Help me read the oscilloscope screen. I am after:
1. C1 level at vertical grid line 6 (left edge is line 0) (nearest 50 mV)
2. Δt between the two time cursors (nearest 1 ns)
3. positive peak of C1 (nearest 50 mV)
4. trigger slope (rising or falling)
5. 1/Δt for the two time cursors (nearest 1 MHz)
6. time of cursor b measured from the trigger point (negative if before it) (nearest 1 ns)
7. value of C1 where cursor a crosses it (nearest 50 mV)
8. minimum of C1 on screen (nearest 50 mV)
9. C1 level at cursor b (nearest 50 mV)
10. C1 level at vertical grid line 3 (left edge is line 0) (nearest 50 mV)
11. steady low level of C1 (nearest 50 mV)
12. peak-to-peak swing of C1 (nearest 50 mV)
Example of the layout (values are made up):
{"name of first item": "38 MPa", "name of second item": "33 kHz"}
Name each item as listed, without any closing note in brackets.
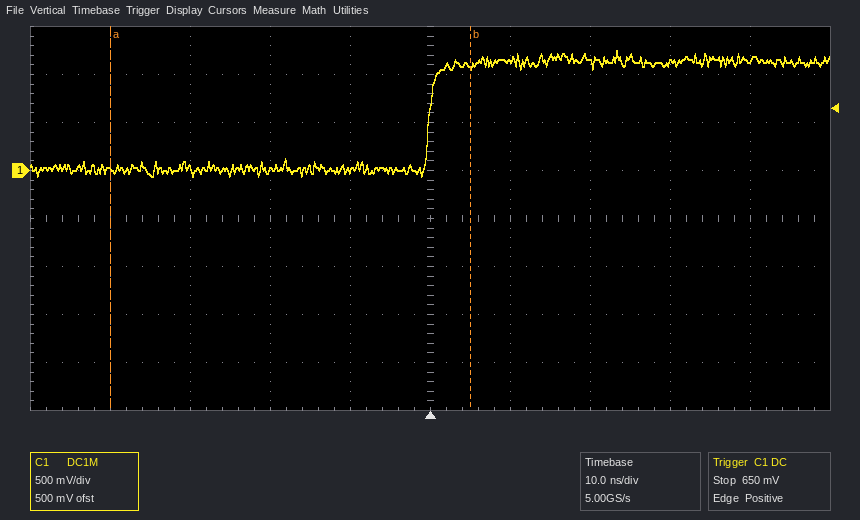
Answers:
{"C1 level at vertical grid line 6 (left edge is line 0)": "1.15 V", "Δt between the two time cursors": "45 ns", "positive peak of C1": "1.25 V", "trigger slope": "rising", "1/Δt for the two time cursors": "22 MHz", "time of cursor b measured from the trigger point (negative if before it)": "+5 ns", "value of C1 where cursor a crosses it": "0 mV", "minimum of C1 on screen": "-50 mV", "C1 level at cursor b": "1.10 V", "C1 level at vertical grid line 3 (left edge is line 0)": "0 mV", "steady low level of C1": "0 mV", "peak-to-peak swing of C1": "1.30 V"}
